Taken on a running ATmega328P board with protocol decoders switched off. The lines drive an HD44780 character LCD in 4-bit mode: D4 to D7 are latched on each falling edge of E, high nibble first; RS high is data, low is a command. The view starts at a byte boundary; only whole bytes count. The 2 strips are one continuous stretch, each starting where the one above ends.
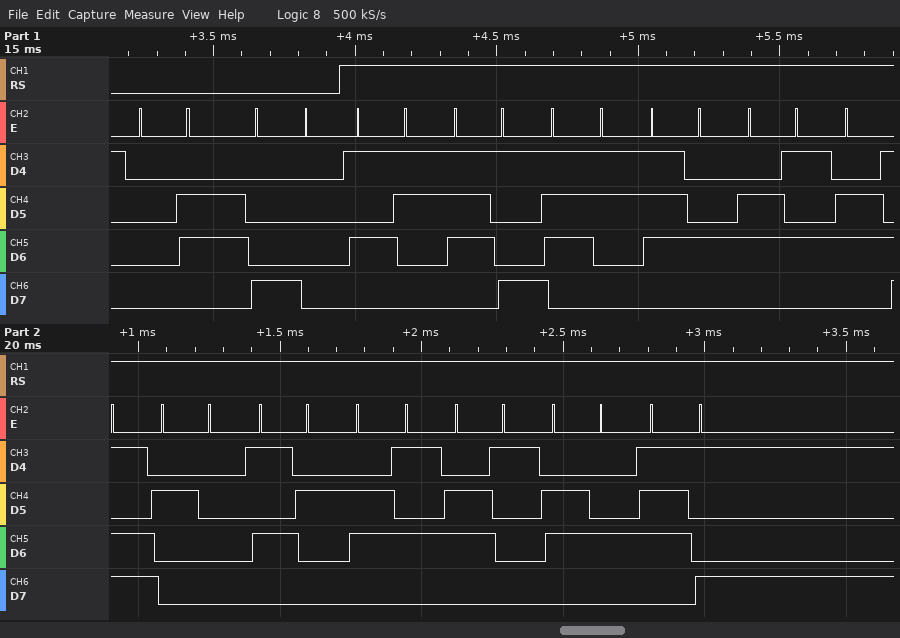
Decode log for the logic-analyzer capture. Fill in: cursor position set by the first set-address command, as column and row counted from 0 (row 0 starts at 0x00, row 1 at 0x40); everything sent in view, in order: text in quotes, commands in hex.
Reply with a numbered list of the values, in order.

1. column 0, row 0
2. 0x06 0x80 "System Ready"
